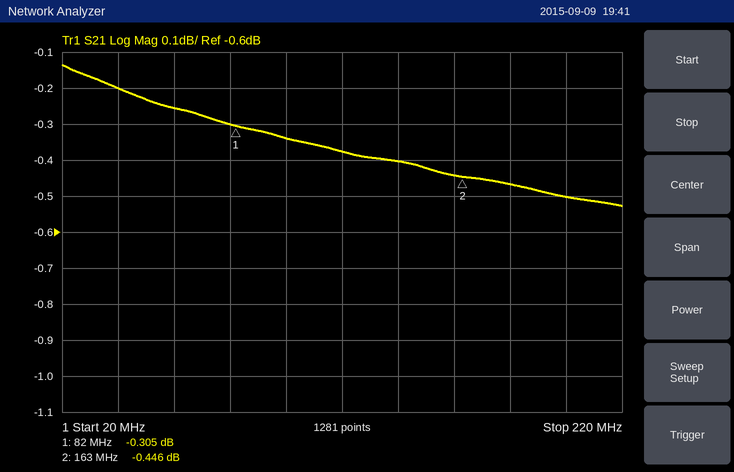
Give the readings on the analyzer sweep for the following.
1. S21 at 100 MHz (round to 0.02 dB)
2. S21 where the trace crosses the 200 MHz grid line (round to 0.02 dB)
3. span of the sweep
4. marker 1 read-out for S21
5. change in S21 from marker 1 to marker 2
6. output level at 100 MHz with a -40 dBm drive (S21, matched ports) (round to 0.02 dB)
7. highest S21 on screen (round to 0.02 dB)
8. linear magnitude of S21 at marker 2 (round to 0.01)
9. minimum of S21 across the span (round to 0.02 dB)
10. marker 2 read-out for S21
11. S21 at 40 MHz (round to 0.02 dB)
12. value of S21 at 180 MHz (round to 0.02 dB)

-0.34 dB
-0.50 dB
200 MHz
-0.305 dB
-0.141 dB
-40.34 dBm
-0.14 dB
0.95
-0.52 dB
-0.446 dB
-0.20 dB
-0.46 dB
